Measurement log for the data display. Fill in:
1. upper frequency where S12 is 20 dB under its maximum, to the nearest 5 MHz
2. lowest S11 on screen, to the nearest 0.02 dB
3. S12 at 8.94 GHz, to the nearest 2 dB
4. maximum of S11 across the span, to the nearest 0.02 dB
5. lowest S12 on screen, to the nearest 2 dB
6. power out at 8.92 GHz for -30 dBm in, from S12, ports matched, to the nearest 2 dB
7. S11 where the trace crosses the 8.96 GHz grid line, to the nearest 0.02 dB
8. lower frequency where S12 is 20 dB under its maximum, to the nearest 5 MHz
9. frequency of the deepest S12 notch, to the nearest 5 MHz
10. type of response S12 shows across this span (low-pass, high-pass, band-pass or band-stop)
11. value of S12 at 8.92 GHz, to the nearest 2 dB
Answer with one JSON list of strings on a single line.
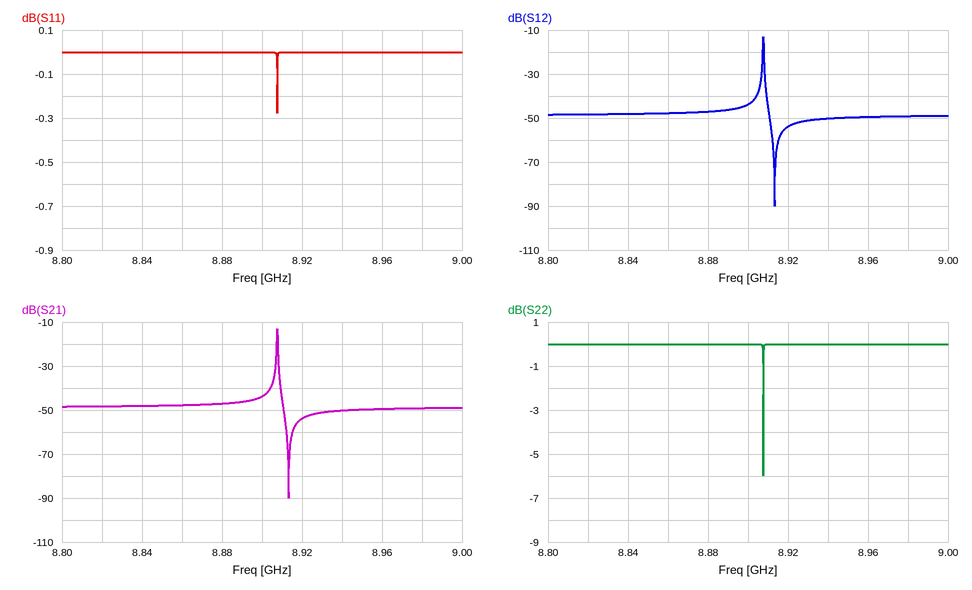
["8.910 GHz", "-0.28 dB", "-50 dB", "0.00 dB", "-90 dB", "-84 dBm", "0.00 dB", "8.905 GHz", "8.915 GHz", "band-pass", "-54 dB"]
